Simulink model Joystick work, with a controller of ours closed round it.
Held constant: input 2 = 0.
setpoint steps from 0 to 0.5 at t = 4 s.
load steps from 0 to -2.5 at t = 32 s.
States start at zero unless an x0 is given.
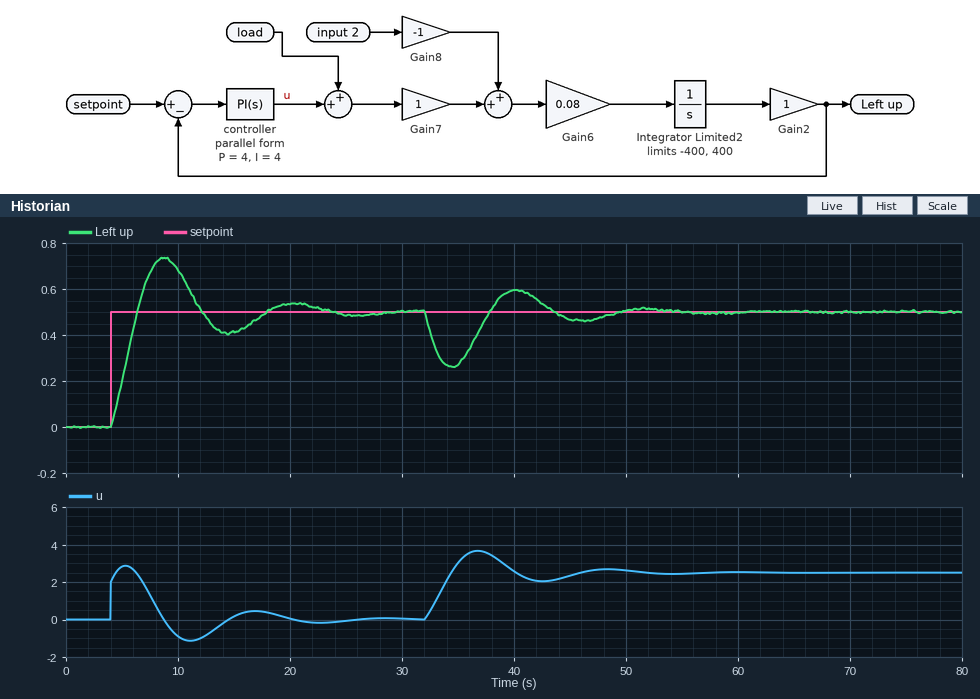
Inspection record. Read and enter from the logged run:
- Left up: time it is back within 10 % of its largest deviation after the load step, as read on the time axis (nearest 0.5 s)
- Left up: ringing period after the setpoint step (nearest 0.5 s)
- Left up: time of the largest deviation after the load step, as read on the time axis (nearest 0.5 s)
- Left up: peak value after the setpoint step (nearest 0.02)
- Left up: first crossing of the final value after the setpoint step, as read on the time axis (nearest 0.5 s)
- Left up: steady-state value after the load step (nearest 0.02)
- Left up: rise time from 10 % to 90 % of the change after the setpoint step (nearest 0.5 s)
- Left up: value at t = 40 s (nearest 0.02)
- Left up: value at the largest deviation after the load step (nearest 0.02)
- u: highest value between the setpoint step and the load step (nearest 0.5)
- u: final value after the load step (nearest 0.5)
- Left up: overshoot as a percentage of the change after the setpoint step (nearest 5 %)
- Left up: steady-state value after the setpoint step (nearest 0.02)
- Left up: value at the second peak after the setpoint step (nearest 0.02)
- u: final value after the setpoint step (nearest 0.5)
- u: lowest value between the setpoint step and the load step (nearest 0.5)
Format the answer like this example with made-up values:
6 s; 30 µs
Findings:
47.5 s; 11.5 s; 34.5 s; 0.74; 6.5 s; 0.50; 2.0 s; 0.60; 0.26; 3.0; 2.5; 45 %; 0.50; 0.54; 0.0; -1.0
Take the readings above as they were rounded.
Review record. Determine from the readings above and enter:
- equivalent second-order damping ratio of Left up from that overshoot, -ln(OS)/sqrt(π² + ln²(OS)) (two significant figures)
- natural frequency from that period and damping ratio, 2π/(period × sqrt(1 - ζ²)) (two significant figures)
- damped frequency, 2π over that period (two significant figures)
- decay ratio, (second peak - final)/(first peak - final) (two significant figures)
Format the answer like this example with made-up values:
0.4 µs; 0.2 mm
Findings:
0.25; 0.56 rad/s; 0.55 rad/s; 0.17
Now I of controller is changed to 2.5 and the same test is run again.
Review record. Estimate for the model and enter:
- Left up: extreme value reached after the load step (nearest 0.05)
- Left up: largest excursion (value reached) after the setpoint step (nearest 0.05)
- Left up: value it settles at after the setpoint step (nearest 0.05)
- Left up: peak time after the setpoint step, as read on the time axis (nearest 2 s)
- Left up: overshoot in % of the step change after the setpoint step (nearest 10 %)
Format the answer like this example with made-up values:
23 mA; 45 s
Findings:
0.20; 0.70; 0.50; 10 s; 40 %
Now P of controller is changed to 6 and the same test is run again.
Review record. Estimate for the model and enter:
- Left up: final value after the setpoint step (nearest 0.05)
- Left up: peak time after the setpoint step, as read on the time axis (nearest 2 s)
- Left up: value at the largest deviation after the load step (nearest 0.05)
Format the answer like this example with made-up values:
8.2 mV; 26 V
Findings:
0.50; 8 s; 0.30
